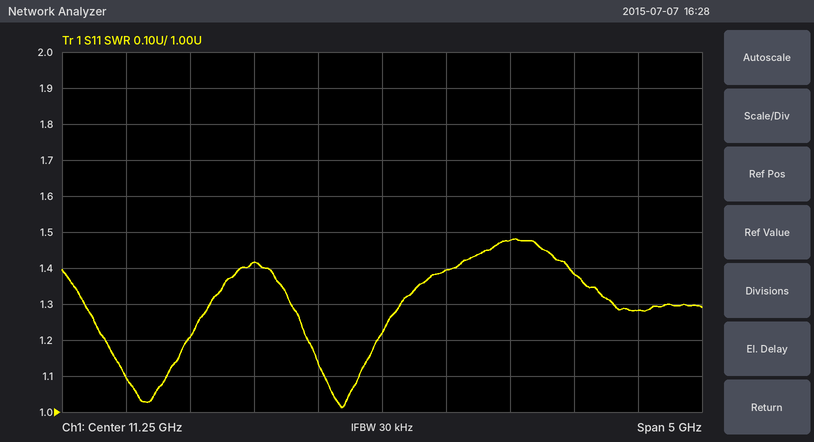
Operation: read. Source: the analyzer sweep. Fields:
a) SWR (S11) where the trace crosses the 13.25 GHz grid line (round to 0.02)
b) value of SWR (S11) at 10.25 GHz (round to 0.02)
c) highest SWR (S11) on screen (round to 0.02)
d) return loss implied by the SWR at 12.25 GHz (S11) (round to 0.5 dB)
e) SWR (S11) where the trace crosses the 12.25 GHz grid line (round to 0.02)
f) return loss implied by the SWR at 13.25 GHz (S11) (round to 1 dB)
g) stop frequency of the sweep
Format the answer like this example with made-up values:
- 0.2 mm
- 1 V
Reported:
- 1.28
- 1.42
- 1.48
- 14.5 dB
- 1.48
- 18 dB
- 13.75 GHz
